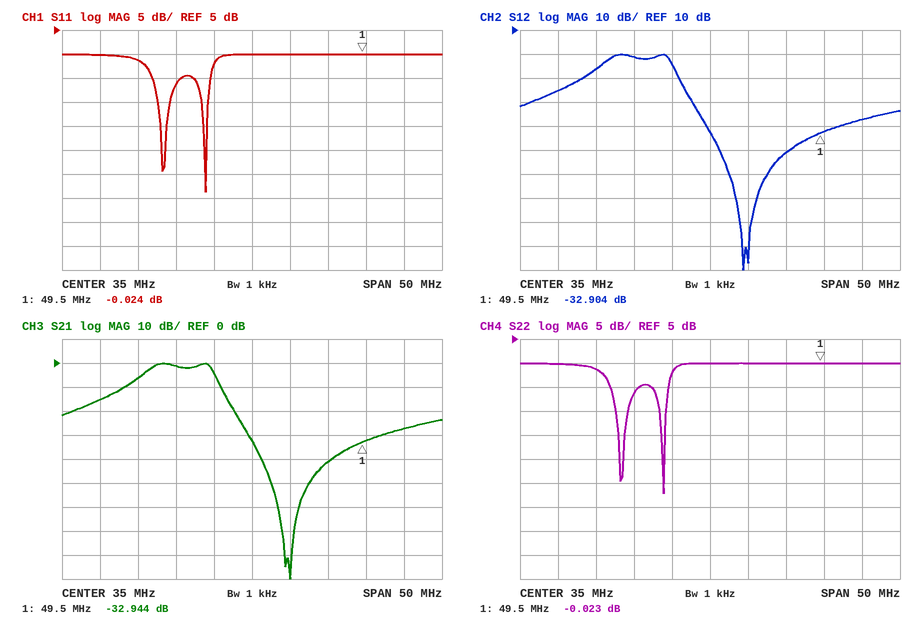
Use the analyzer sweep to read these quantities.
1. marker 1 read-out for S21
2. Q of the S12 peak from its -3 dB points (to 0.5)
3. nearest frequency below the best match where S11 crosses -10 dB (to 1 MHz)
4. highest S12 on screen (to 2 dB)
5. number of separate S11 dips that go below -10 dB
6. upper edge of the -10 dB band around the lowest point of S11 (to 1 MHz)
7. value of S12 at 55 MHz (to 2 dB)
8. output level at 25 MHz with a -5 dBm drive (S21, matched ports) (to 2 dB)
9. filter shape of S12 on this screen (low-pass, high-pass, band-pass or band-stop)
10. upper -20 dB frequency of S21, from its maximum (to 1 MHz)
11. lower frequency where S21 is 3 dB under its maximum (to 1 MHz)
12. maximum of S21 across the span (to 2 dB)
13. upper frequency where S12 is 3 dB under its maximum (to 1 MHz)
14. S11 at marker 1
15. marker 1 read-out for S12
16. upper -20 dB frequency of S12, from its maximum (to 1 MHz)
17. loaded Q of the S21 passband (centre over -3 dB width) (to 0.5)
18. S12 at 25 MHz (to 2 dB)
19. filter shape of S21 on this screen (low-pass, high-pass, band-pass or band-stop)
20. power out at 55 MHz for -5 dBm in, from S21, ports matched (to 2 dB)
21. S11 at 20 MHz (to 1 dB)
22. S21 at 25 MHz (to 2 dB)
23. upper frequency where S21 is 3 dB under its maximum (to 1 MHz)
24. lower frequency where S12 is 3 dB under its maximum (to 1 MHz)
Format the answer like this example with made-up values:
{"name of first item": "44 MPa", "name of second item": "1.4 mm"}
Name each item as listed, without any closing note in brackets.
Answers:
{"marker 1 read-out for S21": "-32.944 dB", "Q of the S12 peak from its -3 dB points": "3.0", "nearest frequency below the best match where S11 crosses -10 dB": "28 MHz", "highest S12 on screen": "0 dB", "number of separate S11 dips that go below -10 dB": "2", "upper edge of the -10 dB band around the lowest point of S11": "29 MHz", "value of S12 at 55 MHz": "-28 dB", "output level at 25 MHz with a -5 dBm drive (S21, matched ports)": "-6 dBm", "filter shape of S12 on this screen": "band-pass", "upper -20 dB frequency of S21, from its maximum": "33 MHz", "lower frequency where S21 is 3 dB under its maximum": "21 MHz", "maximum of S21 across the span": "0 dB", "upper frequency where S12 is 3 dB under its maximum": "30 MHz", "S11 at marker 1": "-0.024 dB", "marker 1 read-out for S12": "-32.904 dB", "upper -20 dB frequency of S12, from its maximum": "33 MHz", "loaded Q of the S21 passband (centre over -3 dB width)": "3.0", "S12 at 25 MHz": "-2 dB", "filter shape of S21 on this screen": "band-pass", "power out at 55 MHz for -5 dBm in, from S21, ports matched": "-32 dBm", "S11 at 20 MHz": "-1 dB", "S21 at 25 MHz": "-2 dB", "upper frequency where S21 is 3 dB under its maximum": "30 MHz", "lower frequency where S12 is 3 dB under its maximum": "21 MHz"}
